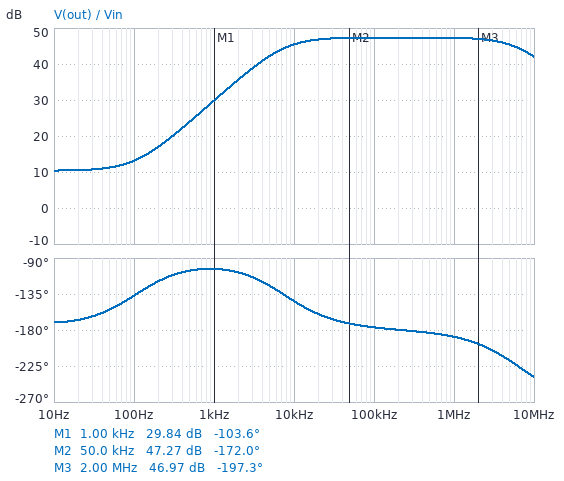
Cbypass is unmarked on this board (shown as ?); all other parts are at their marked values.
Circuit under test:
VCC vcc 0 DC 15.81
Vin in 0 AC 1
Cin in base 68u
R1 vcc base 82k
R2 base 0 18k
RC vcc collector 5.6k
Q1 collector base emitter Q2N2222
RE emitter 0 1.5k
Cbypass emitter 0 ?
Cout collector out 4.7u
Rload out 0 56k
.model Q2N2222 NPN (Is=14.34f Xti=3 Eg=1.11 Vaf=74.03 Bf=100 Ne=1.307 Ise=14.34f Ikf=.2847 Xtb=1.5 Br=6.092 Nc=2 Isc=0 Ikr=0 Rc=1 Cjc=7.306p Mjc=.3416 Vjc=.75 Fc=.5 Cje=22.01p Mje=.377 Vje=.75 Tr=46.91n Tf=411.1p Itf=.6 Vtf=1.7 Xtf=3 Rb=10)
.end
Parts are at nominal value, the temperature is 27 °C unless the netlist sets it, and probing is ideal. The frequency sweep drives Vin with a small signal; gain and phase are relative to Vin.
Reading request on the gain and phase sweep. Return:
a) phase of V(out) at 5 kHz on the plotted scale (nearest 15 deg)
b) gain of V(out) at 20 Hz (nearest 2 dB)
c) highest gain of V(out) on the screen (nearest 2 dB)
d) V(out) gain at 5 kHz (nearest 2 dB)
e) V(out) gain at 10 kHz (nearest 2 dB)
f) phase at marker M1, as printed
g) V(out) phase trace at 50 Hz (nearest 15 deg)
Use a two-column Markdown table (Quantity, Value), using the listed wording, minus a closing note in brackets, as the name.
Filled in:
| Quantity | Value |
|---|---|
| phase of V(out) at 5 kHz on the plotted scale | -120 deg |
| gain of V(out) at 20 Hz | 10 dB |
| highest gain of V(out) on the screen | 48 dB |
| V(out) gain at 5 kHz | 42 dB |
| V(out) gain at 10 kHz | 46 dB |
| phase at marker M1, as printed | -103.6 deg |
| V(out) phase trace at 50 Hz | -150 deg |
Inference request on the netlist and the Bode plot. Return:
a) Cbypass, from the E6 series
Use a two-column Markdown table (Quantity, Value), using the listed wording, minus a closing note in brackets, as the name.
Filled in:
| Quantity | Value |
|---|---|
| Cbypass, from the E6 series | 1 µF |
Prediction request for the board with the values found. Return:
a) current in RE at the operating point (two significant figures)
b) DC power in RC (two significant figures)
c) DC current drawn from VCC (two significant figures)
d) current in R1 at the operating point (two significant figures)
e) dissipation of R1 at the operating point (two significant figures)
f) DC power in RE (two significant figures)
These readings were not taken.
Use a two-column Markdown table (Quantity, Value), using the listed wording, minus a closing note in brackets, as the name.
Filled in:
| Quantity | Value |
|---|---|
| current in RE at the operating point | 1.3 mA |
| DC power in RC | 9.4 mW |
| DC current drawn from VCC | 1.5 mA |
| current in R1 at the operating point | 160 µA |
| dissipation of R1 at the operating point | 2.1 mW |
| DC power in RE | 2.6 mW |
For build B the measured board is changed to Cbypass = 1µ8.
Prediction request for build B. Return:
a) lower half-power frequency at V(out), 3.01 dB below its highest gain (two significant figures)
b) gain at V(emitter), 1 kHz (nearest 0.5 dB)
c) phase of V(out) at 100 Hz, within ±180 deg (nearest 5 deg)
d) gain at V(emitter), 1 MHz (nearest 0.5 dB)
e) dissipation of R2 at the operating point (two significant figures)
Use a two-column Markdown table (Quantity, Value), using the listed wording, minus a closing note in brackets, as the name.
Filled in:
| Quantity | Value |
|---|---|
| lower half-power frequency at V(out), 3.01 dB below its highest gain | 4.2 kHz |
| gain at V(emitter), 1 kHz | -0.5 dB |
| phase of V(out) at 100 Hz, within ±180 deg | -120 deg |
| gain at V(emitter), 1 MHz | -48.0 dB |
| dissipation of R2 at the operating point | 380 µW |
